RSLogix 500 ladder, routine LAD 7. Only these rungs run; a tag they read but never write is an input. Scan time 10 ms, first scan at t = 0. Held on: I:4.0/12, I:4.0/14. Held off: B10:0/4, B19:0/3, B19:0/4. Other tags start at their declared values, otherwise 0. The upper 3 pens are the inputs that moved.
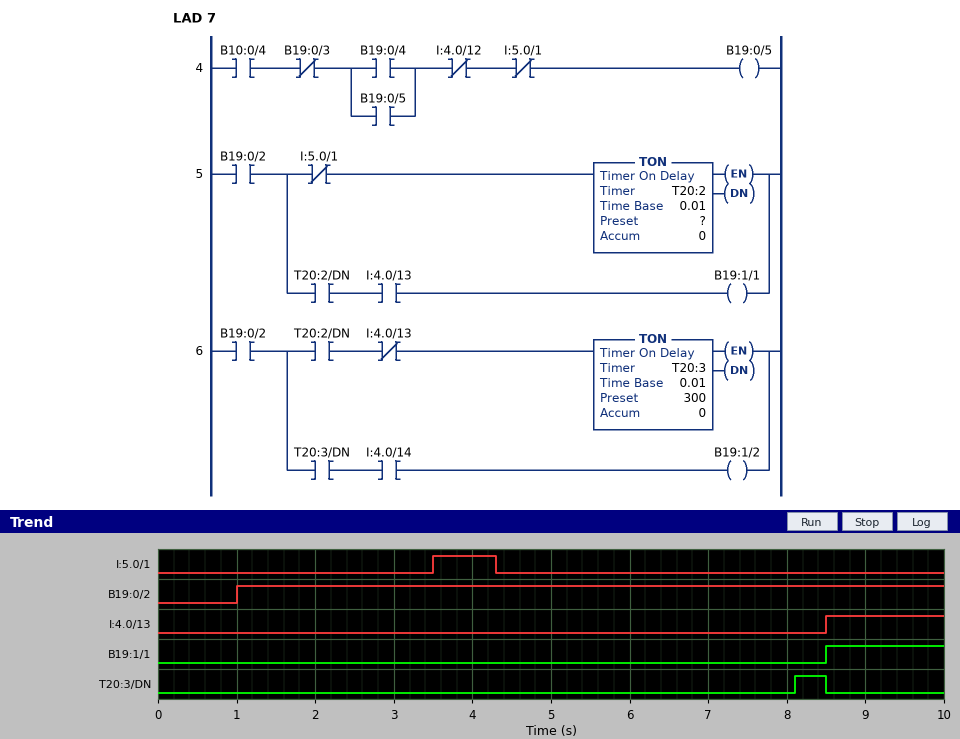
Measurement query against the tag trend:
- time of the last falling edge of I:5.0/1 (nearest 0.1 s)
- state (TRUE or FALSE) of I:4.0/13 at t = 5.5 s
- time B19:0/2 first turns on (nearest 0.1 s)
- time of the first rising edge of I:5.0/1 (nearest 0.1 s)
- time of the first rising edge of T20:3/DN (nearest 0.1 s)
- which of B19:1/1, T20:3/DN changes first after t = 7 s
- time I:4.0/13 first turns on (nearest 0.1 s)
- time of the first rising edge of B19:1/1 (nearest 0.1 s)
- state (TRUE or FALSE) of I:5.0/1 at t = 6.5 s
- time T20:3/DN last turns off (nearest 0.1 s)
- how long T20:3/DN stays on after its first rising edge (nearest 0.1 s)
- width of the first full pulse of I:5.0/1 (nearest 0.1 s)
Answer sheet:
4.3 s
FALSE
1.0 s
3.5 s
8.1 s
T20:3/DN
8.5 s
8.5 s
FALSE
8.5 s
0.4 s
0.8 s
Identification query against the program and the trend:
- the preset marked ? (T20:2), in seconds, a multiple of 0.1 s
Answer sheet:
0.8 s
